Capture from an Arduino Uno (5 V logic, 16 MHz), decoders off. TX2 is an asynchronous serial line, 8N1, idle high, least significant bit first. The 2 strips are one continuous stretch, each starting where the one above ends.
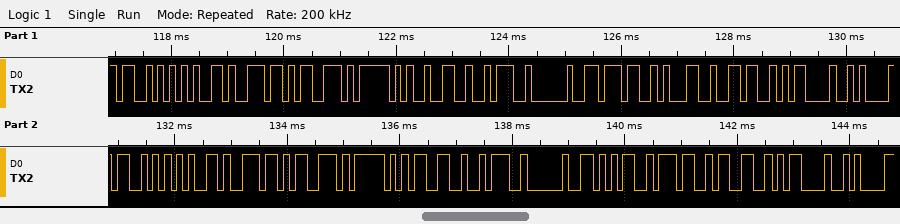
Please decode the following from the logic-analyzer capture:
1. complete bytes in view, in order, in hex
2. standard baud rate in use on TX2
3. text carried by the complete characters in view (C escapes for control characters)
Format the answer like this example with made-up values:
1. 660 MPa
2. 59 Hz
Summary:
1. 53 65 6E 73 5F 32 3A 20 37 31 36 0D 0A 53 65 6E 73 5F 33 3A 20 35 37 33 0D 0A
2. 9600 baud
3. "Sens_2: 716\r\nSens_3: 573\r\n"
